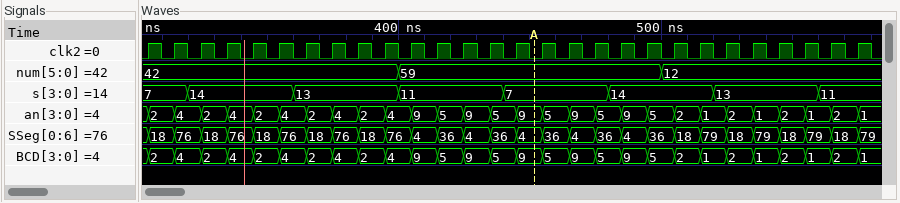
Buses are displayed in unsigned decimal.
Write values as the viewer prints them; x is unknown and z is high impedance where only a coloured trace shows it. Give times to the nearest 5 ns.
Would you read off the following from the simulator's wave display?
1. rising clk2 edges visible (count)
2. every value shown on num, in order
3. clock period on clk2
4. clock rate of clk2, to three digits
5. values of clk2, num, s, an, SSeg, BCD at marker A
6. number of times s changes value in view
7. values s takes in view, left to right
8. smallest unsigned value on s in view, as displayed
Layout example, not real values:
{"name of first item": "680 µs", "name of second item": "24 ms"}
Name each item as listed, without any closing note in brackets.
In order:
{"rising clk2 edges visible": "28", "every value shown on num, in order": "42, 59, 12", "clock period on clk2": "10 ns", "clock rate of clk2, to three digits": "100 MHz", "values of clk2, num, s, an, SSeg, BCD at marker A": "clk2=0, num=59, s=7, an=9, SSeg=4, BCD=9", "number of times s changes value in view": "7", "values s takes in view, left to right": "7, 14, 13, 11, 7, 14, 13, 11", "smallest unsigned value on s in view, as displayed": "7"}
